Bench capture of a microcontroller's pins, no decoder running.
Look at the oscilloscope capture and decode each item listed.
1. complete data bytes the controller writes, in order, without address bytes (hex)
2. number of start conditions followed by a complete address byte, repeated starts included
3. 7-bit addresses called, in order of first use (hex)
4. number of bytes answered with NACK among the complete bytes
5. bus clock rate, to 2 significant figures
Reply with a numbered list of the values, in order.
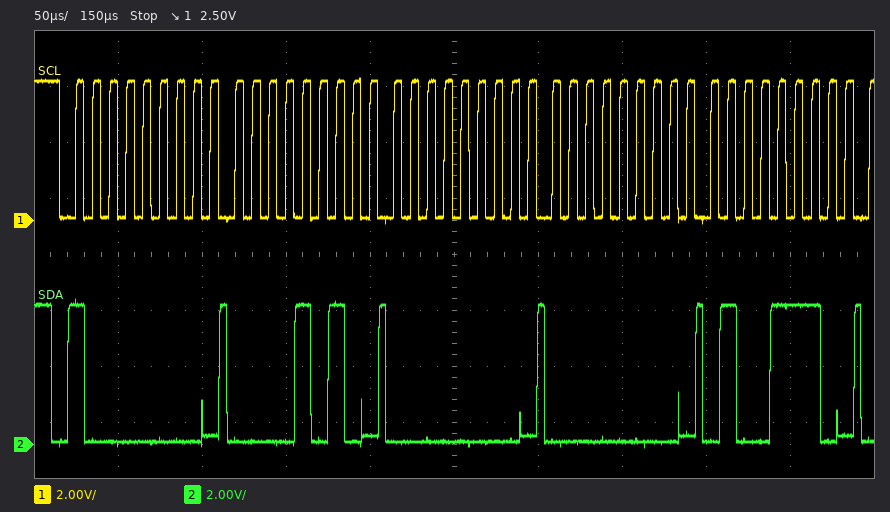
1. 0A 00 00 4E
2. 1
3. 0x40
4. 0
5. 100 kHz
